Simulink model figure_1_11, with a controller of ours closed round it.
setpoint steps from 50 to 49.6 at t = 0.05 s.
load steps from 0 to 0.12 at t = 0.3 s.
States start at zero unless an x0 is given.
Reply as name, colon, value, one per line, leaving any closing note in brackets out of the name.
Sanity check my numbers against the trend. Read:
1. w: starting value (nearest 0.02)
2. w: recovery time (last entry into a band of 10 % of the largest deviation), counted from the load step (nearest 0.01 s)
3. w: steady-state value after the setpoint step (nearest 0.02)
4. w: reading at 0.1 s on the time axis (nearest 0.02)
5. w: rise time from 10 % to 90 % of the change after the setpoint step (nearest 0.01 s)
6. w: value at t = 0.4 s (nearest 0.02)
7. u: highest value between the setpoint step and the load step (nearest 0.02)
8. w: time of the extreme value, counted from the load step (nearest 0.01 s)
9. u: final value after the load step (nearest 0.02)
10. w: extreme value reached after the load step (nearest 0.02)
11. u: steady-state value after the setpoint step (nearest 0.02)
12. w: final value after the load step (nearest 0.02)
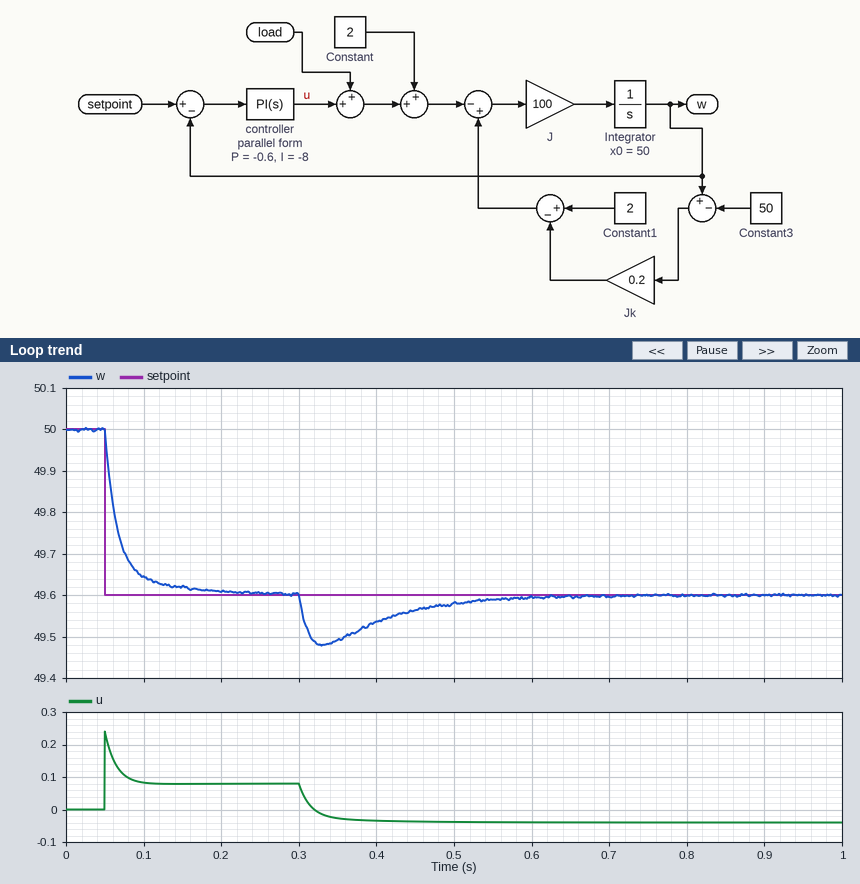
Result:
w: starting value: 50.00
w: recovery time (last entry into a band of 10 % of the largest deviation), counted from the load step: 0.24 s
w: steady-state value after the setpoint step: 49.60
w: reading at 0.1 s on the time axis: 49.64
w: rise time from 10 % to 90 % of the change after the setpoint step: 0.05 s
w: value at t = 0.4 s: 49.54
u: highest value between the setpoint step and the load step: 0.24
w: time of the extreme value, counted from the load step: 0.03 s
u: final value after the load step: -0.04
w: extreme value reached after the load step: 49.48
u: steady-state value after the setpoint step: 0.08
w: final value after the load step: 49.60
